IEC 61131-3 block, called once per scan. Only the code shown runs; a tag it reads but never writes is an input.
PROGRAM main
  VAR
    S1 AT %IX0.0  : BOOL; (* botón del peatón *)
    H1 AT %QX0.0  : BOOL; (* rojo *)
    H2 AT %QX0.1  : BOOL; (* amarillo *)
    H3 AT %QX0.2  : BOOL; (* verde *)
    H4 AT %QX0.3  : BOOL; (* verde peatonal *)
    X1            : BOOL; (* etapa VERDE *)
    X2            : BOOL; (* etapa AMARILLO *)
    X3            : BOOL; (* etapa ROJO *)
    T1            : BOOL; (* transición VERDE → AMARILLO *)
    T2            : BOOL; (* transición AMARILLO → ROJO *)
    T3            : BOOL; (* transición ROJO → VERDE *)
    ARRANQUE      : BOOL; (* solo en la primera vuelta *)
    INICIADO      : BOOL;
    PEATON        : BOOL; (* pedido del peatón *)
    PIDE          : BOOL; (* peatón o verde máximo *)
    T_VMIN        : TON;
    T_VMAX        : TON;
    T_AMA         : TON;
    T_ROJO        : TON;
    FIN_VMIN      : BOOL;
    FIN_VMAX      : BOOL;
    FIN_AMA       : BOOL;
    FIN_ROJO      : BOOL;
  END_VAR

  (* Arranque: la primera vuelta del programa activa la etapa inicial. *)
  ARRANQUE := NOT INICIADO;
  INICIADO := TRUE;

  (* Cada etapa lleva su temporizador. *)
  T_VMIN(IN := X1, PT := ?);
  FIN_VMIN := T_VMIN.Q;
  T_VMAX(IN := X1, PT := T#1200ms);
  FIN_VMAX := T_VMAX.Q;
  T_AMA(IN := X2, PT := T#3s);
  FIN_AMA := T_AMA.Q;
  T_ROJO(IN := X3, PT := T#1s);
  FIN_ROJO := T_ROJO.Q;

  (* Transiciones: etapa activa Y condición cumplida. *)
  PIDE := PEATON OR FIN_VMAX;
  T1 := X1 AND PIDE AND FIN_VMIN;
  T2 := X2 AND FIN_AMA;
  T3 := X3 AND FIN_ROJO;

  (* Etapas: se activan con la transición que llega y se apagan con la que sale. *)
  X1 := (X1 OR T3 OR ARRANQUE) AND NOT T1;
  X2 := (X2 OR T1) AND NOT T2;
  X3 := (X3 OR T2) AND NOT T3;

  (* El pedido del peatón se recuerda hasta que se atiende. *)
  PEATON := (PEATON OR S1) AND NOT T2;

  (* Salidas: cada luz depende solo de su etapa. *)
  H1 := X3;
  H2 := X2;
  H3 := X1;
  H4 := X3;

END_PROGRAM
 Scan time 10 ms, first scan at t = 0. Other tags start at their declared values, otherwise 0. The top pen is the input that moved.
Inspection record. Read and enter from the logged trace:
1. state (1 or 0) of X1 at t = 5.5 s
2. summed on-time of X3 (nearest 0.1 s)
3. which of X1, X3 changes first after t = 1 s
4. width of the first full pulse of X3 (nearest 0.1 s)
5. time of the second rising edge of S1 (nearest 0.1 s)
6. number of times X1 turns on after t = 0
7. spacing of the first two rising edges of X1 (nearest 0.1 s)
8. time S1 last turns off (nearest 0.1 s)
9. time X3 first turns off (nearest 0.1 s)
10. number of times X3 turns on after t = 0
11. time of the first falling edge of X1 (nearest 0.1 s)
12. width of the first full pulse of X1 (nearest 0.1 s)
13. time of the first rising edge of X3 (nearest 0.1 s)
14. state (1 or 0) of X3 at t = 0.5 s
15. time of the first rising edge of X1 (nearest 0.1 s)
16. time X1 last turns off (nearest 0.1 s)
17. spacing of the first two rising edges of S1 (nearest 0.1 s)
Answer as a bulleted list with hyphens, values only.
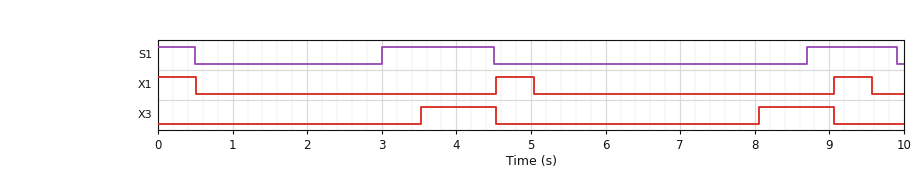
- 0
- 2.0 s
- X3
- 1.0 s
- 8.7 s
- 2
- 4.5 s
- 9.9 s
- 4.5 s
- 2
- 0.5 s
- 0.5 s
- 3.5 s
- 0
- 4.5 s
- 9.6 s
- 5.7 s
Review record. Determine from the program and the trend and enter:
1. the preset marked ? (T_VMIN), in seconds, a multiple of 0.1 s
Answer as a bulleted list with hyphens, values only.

- 0.5 s
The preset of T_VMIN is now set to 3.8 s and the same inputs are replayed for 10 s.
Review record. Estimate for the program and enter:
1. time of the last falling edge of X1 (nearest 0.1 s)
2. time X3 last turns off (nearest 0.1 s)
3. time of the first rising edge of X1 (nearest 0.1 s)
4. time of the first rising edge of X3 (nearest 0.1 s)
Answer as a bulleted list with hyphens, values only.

- 3.8 s
- 7.8 s
- 7.8 s
- 6.8 s
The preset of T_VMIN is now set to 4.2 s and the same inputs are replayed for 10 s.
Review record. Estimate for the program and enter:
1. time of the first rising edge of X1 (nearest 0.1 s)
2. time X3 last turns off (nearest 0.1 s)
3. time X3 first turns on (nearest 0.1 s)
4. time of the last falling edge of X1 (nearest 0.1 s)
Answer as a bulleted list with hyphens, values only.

- 8.2 s
- 8.2 s
- 7.2 s
- 4.2 s
